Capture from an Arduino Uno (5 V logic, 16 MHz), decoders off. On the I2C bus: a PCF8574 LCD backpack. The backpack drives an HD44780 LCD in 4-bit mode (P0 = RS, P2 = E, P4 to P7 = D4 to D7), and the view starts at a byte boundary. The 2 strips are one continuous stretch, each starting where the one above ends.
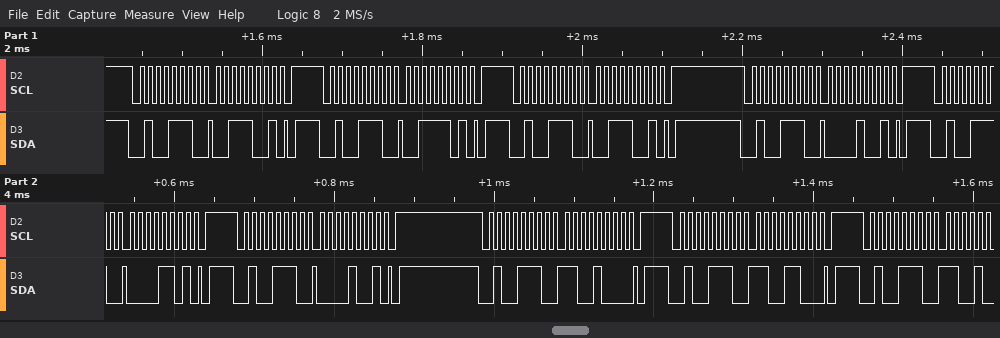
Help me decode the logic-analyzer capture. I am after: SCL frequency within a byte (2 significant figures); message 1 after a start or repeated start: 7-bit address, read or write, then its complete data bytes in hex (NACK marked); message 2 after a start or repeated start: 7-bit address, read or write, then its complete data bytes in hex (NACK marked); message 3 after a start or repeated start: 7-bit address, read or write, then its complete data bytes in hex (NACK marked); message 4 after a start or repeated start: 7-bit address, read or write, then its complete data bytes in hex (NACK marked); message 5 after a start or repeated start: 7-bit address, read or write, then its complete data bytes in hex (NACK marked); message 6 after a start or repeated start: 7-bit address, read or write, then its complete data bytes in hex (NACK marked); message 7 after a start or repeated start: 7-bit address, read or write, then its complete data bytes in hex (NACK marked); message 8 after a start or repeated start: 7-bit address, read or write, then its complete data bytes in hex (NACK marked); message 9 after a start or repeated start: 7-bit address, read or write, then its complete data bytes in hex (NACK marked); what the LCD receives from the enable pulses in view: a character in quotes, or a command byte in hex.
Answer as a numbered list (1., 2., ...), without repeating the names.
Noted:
1. 100 kHz
2. 0x27 write: 39
3. 0x27 write: 3D
4. 0x27 write: 39
5. 0x27 write: 09
6. 0x27 write: 0D
7. 0x27 write: 09
8. 0x27 write: C8
9. 0x27 write: CC
10. 0x27 write
11. '0'
